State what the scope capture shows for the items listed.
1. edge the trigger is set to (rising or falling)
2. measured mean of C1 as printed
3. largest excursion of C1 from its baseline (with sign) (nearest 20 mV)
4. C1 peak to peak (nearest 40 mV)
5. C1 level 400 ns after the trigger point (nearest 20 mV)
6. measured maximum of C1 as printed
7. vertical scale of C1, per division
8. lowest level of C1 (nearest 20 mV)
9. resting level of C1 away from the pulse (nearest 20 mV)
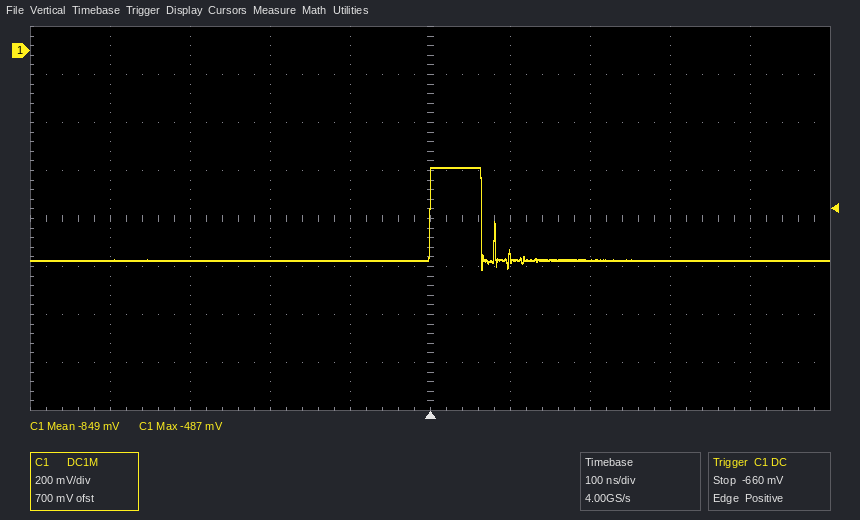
rising
-849 mV
+380 mV
440 mV
-880 mV
-487 mV
200 mV
-920 mV
-880 mV
